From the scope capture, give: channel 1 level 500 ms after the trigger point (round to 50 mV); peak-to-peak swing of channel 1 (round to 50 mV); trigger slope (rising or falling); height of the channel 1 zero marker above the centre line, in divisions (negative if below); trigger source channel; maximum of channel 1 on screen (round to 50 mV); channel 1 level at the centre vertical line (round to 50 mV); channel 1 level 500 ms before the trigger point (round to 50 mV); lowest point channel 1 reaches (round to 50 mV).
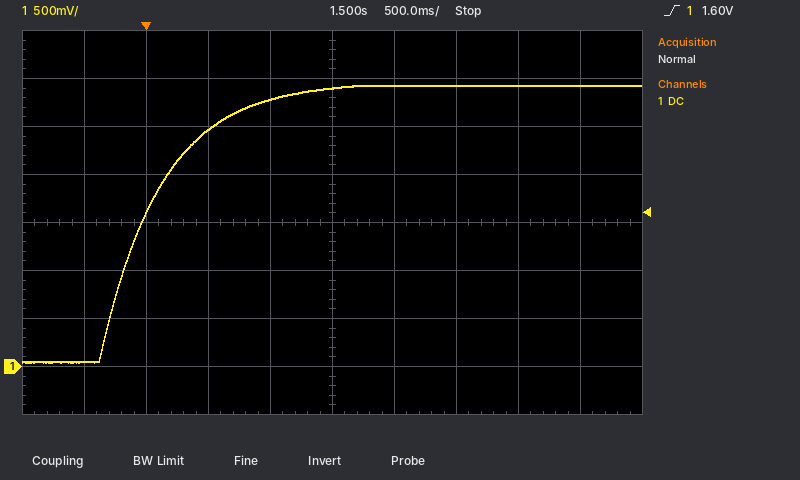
2.45 V
2.90 V
rising
-3.0 div
channel 1
2.95 V
2.90 V
50 mV
50 mV
